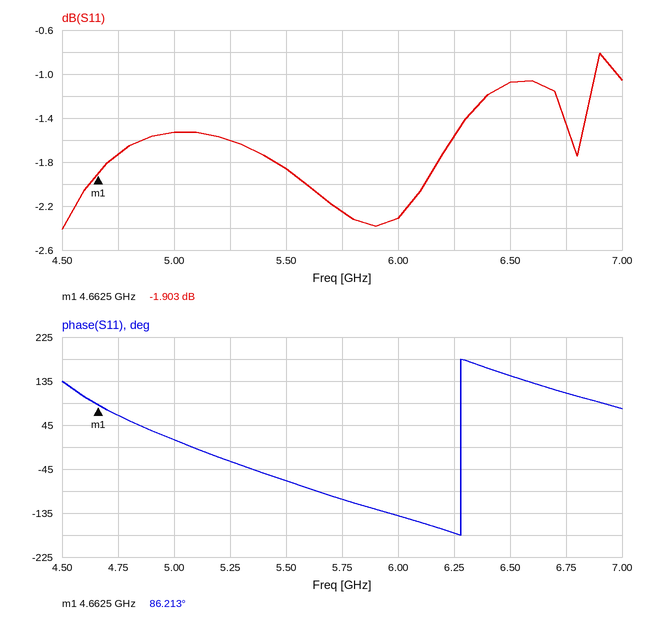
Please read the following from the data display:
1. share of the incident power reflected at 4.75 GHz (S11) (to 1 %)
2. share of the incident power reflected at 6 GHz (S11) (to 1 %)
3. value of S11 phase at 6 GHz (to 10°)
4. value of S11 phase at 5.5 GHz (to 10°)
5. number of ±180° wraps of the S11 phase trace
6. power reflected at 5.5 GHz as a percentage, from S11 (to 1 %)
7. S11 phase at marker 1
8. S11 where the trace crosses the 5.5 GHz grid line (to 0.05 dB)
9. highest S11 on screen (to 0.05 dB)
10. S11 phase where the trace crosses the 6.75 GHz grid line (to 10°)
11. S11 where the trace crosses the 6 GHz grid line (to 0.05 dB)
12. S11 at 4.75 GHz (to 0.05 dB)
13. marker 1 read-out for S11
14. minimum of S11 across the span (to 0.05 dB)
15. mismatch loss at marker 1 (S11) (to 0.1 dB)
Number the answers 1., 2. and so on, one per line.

1. 67 %
2. 59 %
3. -140°
4. -70°
5. 1
6. 65 %
7. 86.213°
8. -1.85 dB
9. -0.80 dB
10. 110°
11. -2.30 dB
12. -1.75 dB
13. -1.903 dB
14. -2.40 dB
15. 4.5 dB
